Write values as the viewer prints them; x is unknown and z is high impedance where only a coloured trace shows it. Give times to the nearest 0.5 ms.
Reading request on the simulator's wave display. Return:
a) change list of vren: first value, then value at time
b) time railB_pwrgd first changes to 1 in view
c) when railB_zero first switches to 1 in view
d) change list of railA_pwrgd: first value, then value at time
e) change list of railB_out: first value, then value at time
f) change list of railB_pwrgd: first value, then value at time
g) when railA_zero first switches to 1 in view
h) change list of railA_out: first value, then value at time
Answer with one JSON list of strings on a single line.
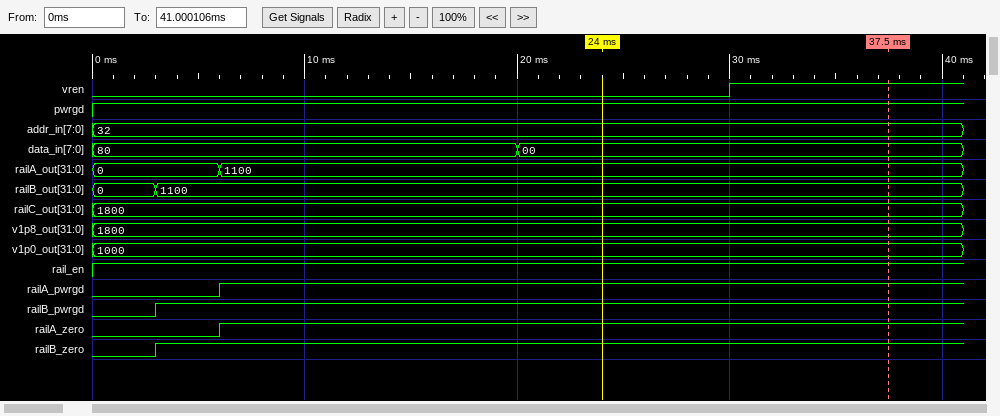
["0, 1 at 30 ms", "3 ms", "3 ms", "0, 1 at 6 ms", "0, 1100 at 3 ms", "0, 1 at 3 ms", "6 ms", "0, 1100 at 6 ms"]
